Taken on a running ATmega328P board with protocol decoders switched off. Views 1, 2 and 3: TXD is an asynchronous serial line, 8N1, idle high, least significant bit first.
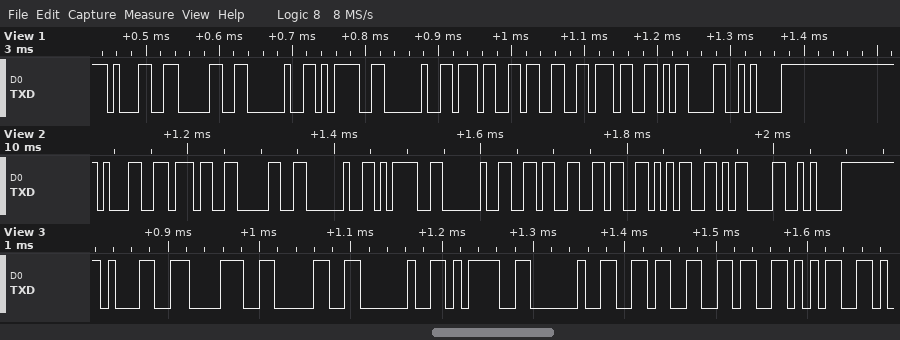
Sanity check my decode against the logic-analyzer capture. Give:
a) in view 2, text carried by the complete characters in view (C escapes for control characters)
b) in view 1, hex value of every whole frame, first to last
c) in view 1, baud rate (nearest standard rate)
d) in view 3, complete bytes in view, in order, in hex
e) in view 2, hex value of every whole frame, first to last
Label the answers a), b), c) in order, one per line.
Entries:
a) "170 = 665\r\n"
b) 31 30 20 3D 20 37 33 37 0D 0A
c) 115200 baud
d) 0x31 0x38 0x30 0x20 0x3D 0x20 0x36 0x36 0x35
e) 31 37 30 20 3D 20 36 36 35 0D 0A
